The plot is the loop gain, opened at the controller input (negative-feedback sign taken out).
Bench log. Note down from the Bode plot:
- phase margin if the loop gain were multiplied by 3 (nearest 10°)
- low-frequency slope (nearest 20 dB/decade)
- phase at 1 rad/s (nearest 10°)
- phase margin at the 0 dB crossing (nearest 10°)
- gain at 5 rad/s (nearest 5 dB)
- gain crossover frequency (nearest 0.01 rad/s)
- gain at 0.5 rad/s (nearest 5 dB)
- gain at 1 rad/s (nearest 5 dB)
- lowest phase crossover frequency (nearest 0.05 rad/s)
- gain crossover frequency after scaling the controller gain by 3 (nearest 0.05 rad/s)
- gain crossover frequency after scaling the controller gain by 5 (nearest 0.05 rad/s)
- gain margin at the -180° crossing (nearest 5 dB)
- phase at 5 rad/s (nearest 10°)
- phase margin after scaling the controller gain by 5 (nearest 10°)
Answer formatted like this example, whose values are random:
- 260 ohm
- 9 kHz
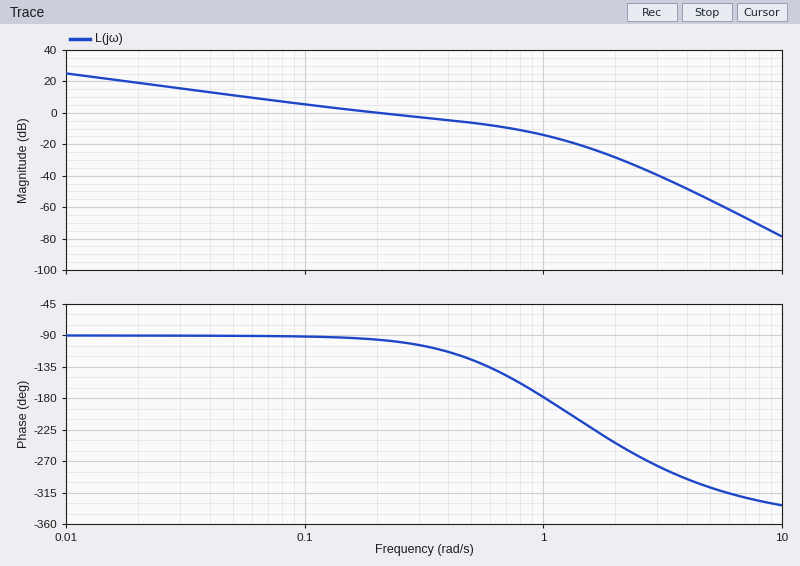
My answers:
- 30°
- -20 dB/decade
- -180°
- 80°
- -55 dB
- 0.20 rad/s
- -5 dB
- -15 dB
- 1.00 rad/s
- 0.70 rad/s
- 1.00 rad/s
- 15 dB
- -310°
- 0°
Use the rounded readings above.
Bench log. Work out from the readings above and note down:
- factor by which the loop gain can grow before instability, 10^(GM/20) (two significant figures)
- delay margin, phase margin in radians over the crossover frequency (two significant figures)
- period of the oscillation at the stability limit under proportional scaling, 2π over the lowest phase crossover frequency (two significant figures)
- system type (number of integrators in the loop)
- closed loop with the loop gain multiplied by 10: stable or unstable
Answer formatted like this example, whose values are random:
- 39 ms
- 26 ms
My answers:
- 5.6
- 7.0 s
- 6.3 s
- 1
- unstable
